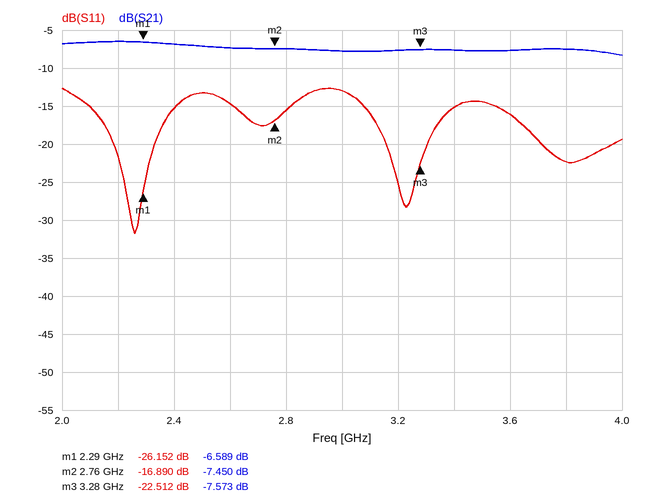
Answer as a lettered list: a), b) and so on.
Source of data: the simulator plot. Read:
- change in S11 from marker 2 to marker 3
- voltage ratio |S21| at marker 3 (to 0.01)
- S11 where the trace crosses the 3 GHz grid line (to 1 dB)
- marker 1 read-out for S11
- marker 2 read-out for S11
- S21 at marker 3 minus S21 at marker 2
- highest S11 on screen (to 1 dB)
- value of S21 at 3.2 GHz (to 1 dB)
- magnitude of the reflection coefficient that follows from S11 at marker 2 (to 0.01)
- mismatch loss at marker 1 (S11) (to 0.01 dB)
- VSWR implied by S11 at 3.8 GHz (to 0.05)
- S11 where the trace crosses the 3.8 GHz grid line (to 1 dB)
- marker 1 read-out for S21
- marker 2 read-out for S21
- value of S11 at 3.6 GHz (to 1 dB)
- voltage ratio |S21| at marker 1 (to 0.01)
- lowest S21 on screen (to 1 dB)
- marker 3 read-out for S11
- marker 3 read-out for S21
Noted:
a) -5.622 dB
b) 0.42
c) -13 dB
d) -26.152 dB
e) -16.890 dB
f) -0.123 dB
g) -13 dB
h) -8 dB
i) 0.14
j) 0.01 dB
k) 1.15
l) -22 dB
m) -6.589 dB
n) -7.450 dB
o) -16 dB
p) 0.47
q) -8 dB
r) -22.512 dB
s) -7.573 dB
